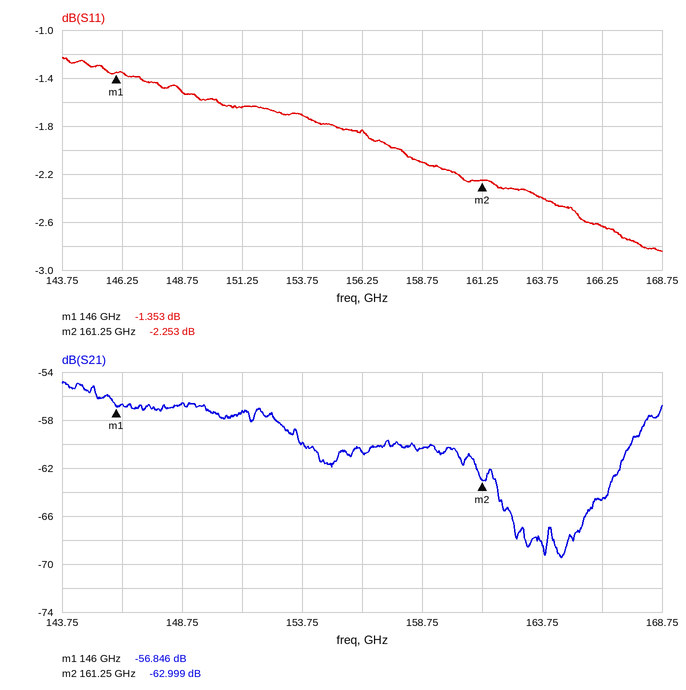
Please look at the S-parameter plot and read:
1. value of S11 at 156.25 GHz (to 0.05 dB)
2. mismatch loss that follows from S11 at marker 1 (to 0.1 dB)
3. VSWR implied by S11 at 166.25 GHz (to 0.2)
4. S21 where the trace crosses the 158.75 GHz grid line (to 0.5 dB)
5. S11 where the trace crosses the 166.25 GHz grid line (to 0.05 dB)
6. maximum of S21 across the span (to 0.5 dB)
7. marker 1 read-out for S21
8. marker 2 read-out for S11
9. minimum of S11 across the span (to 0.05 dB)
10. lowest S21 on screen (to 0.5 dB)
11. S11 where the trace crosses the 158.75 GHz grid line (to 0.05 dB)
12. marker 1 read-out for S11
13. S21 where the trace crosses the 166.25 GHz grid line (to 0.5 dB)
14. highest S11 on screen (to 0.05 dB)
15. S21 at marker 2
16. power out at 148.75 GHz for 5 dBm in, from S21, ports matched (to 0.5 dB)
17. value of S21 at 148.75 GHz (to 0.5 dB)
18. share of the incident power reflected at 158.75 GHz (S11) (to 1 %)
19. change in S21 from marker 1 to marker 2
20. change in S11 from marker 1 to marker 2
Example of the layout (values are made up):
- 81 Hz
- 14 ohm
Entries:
- -1.85 dB
- 5.7 dB
- 6.6
- -60.5 dB
- -2.65 dB
- -55.0 dB
- -56.846 dB
- -2.253 dB
- -2.85 dB
- -69.5 dB
- -2.10 dB
- -1.353 dB
- -64.5 dB
- -1.25 dB
- -62.999 dB
- -51.5 dBm
- -56.5 dB
- 62 %
- -6.153 dB
- -0.900 dB
